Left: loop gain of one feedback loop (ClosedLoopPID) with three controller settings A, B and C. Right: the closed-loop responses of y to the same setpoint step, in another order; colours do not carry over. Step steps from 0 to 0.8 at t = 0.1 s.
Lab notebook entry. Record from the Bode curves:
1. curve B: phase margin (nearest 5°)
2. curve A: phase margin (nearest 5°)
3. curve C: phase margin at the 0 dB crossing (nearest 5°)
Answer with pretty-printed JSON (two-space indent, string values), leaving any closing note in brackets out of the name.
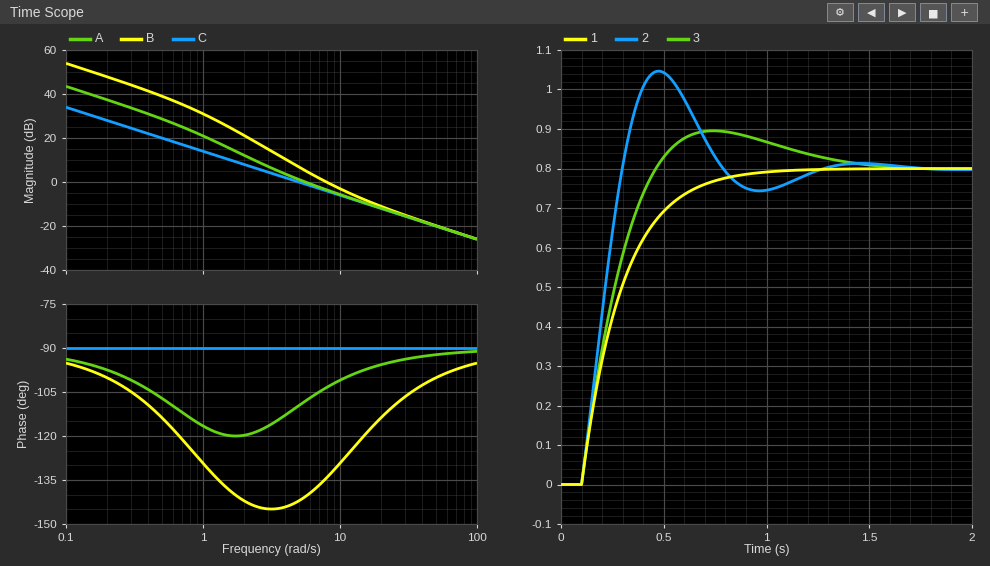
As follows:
{
  "curve B: phase margin": "45°",
  "curve A: phase margin": "70°",
  "curve C: phase margin at the 0 dB crossing": "90°"
}
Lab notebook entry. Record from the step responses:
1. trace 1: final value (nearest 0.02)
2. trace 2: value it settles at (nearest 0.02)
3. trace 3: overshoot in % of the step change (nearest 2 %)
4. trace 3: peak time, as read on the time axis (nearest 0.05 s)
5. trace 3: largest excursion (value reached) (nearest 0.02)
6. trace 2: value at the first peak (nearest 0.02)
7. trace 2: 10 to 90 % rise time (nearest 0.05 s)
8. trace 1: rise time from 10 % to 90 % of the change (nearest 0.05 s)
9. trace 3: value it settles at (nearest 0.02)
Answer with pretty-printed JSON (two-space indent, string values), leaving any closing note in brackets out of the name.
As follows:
{
  "trace 1: final value": "0.80",
  "trace 2: value it settles at": "0.80",
  "trace 3: overshoot in % of the step change": "12 %",
  "trace 3: peak time, as read on the time axis": "0.75 s",
  "trace 3: largest excursion (value reached)": "0.90",
  "trace 2: value at the first peak": "1.04",
  "trace 2: 10 to 90 % rise time": "0.15 s",
  "trace 1: rise time from 10 % to 90 % of the change": "0.45 s",
  "trace 3: value it settles at": "0.80"
}
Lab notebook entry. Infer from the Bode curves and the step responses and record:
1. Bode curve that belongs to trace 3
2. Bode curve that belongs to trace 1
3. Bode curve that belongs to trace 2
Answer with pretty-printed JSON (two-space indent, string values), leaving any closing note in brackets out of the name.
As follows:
{
  "Bode curve that belongs to trace 3": "A",
  "Bode curve that belongs to trace 1": "C",
  "Bode curve that belongs to trace 2": "B"
}
